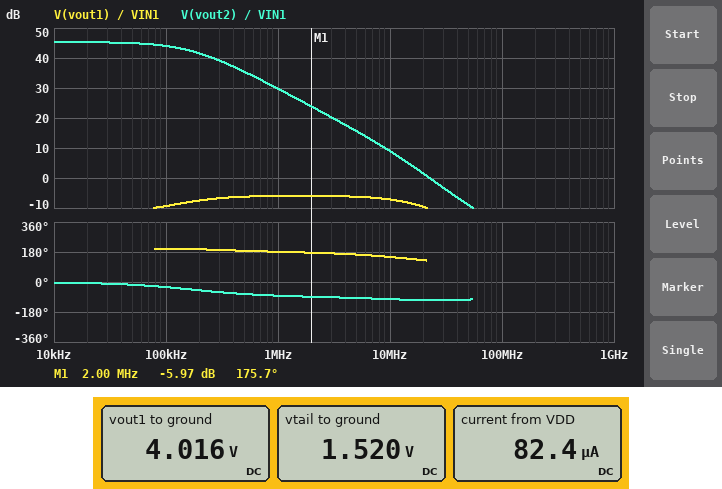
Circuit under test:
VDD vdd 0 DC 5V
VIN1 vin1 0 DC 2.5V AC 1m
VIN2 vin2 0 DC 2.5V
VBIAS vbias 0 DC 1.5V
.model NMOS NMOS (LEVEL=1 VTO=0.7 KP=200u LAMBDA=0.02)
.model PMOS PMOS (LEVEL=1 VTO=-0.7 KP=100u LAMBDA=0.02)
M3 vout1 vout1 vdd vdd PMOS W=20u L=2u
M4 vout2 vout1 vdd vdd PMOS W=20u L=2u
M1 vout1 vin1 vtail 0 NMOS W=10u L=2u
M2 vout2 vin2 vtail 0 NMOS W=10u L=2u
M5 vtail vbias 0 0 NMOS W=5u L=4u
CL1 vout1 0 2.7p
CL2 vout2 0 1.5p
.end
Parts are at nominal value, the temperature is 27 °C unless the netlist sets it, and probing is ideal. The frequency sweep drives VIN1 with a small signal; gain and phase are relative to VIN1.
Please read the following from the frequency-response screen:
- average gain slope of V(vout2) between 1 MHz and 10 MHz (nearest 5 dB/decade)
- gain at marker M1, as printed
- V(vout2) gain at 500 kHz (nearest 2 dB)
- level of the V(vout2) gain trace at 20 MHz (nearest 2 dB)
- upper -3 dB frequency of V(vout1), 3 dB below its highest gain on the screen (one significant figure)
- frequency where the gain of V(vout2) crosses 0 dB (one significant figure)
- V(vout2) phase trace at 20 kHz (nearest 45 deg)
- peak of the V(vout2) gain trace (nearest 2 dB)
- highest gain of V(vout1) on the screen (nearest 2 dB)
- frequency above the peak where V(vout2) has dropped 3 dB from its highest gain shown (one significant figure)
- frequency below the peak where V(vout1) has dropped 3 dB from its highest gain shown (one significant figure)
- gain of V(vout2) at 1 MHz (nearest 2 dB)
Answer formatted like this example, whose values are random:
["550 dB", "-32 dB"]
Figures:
["-20 dB/decade", "-5.97 dB", "36 dB", "2 dB", "20 MHz", "20 MHz", "0 deg", "46 dB", "-6 dB", "200 kHz", "100 kHz", "30 dB"]
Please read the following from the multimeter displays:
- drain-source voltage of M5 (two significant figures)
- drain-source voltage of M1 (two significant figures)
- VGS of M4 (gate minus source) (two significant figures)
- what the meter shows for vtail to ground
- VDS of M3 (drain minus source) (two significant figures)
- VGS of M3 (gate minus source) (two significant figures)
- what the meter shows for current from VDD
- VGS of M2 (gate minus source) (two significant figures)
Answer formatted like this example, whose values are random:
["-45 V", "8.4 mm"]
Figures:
["1.5 V", "2.5 V", "-980 mV", "1.520 V", "-980 mV", "-980 mV", "82.4 µA", "980 mV"]
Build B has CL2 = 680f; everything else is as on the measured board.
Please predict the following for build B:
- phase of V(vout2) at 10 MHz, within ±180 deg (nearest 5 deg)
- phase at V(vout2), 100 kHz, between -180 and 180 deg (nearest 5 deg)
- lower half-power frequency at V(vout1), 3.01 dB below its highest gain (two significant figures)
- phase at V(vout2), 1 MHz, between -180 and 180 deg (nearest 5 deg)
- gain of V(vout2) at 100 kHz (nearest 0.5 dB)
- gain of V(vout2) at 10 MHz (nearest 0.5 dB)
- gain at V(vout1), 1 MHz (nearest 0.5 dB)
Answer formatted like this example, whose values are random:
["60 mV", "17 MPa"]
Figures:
["-100 deg", "-15 deg", "250 kHz", "-70 deg", "45.0 dB", "16.0 dB", "-6.5 dB"]
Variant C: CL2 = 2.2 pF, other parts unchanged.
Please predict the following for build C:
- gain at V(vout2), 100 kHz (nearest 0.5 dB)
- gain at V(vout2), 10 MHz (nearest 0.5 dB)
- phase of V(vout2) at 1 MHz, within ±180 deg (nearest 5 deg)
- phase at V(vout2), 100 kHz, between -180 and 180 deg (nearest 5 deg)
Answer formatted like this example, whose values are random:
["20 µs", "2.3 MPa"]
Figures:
["43.0 dB", "5.5 dB", "-85 deg", "-40 deg"]
